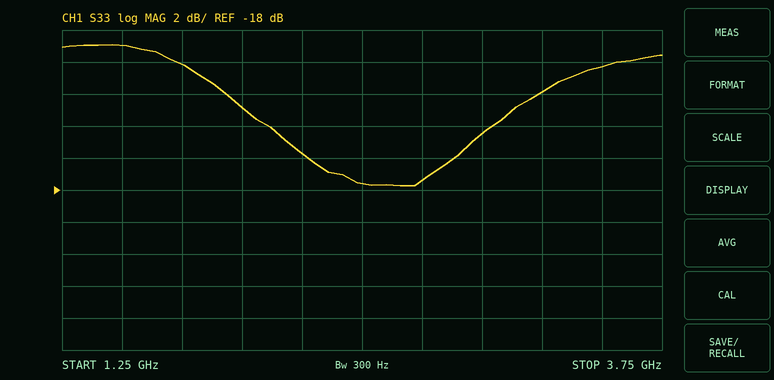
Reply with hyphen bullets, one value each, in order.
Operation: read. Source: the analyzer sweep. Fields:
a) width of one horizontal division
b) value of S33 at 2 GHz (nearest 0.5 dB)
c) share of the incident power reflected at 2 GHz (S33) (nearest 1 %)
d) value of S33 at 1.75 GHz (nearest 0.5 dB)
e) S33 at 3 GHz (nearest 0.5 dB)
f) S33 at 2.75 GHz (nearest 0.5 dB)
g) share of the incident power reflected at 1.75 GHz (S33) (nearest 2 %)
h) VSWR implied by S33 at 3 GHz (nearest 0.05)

- 250 MHz
- -13.0 dB
- 5 %
- -10.0 dB
- -14.5 dB
- -17.5 dB
- 10 %
- 1.45
